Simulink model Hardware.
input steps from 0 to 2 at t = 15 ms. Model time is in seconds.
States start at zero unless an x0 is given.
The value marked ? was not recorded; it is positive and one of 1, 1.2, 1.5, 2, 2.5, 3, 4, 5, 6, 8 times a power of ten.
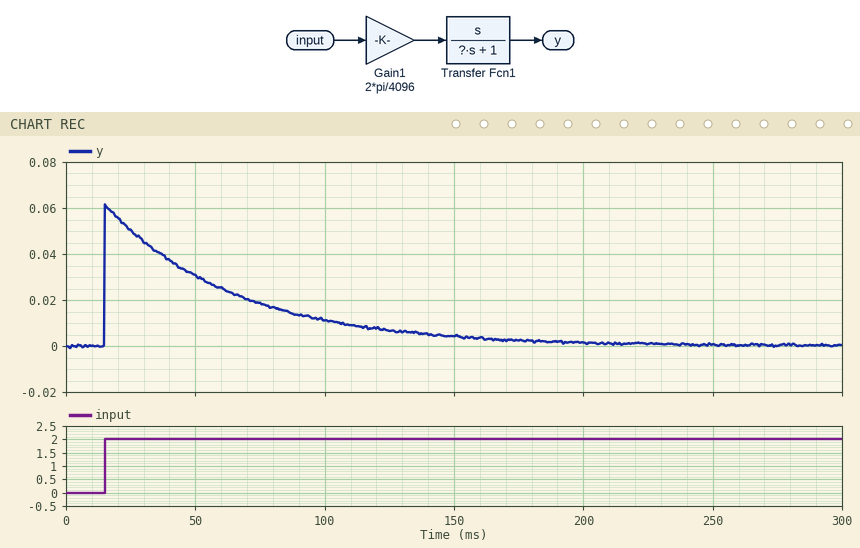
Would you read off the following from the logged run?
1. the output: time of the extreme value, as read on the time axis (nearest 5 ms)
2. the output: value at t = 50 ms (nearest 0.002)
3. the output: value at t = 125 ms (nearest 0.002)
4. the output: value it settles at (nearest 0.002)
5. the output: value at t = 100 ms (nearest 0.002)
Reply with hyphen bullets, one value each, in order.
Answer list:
- 15 ms
- 0.030
- 0.006
- 0.000
- 0.012
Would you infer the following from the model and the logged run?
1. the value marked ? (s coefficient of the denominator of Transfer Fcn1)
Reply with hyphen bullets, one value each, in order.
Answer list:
- 0.05
